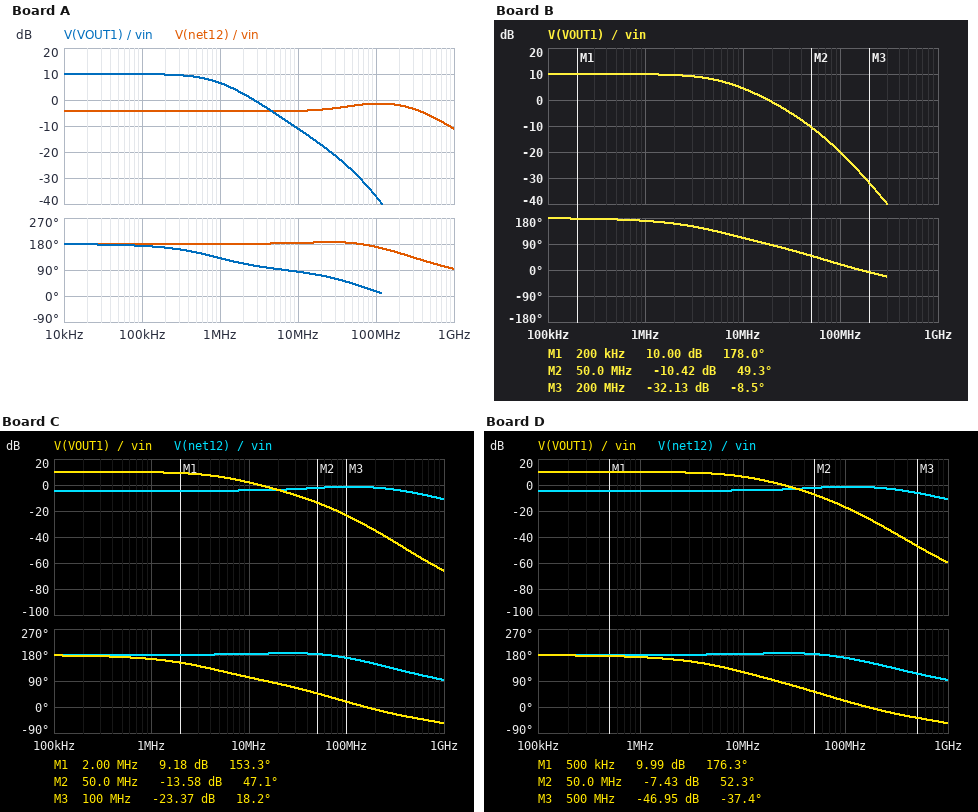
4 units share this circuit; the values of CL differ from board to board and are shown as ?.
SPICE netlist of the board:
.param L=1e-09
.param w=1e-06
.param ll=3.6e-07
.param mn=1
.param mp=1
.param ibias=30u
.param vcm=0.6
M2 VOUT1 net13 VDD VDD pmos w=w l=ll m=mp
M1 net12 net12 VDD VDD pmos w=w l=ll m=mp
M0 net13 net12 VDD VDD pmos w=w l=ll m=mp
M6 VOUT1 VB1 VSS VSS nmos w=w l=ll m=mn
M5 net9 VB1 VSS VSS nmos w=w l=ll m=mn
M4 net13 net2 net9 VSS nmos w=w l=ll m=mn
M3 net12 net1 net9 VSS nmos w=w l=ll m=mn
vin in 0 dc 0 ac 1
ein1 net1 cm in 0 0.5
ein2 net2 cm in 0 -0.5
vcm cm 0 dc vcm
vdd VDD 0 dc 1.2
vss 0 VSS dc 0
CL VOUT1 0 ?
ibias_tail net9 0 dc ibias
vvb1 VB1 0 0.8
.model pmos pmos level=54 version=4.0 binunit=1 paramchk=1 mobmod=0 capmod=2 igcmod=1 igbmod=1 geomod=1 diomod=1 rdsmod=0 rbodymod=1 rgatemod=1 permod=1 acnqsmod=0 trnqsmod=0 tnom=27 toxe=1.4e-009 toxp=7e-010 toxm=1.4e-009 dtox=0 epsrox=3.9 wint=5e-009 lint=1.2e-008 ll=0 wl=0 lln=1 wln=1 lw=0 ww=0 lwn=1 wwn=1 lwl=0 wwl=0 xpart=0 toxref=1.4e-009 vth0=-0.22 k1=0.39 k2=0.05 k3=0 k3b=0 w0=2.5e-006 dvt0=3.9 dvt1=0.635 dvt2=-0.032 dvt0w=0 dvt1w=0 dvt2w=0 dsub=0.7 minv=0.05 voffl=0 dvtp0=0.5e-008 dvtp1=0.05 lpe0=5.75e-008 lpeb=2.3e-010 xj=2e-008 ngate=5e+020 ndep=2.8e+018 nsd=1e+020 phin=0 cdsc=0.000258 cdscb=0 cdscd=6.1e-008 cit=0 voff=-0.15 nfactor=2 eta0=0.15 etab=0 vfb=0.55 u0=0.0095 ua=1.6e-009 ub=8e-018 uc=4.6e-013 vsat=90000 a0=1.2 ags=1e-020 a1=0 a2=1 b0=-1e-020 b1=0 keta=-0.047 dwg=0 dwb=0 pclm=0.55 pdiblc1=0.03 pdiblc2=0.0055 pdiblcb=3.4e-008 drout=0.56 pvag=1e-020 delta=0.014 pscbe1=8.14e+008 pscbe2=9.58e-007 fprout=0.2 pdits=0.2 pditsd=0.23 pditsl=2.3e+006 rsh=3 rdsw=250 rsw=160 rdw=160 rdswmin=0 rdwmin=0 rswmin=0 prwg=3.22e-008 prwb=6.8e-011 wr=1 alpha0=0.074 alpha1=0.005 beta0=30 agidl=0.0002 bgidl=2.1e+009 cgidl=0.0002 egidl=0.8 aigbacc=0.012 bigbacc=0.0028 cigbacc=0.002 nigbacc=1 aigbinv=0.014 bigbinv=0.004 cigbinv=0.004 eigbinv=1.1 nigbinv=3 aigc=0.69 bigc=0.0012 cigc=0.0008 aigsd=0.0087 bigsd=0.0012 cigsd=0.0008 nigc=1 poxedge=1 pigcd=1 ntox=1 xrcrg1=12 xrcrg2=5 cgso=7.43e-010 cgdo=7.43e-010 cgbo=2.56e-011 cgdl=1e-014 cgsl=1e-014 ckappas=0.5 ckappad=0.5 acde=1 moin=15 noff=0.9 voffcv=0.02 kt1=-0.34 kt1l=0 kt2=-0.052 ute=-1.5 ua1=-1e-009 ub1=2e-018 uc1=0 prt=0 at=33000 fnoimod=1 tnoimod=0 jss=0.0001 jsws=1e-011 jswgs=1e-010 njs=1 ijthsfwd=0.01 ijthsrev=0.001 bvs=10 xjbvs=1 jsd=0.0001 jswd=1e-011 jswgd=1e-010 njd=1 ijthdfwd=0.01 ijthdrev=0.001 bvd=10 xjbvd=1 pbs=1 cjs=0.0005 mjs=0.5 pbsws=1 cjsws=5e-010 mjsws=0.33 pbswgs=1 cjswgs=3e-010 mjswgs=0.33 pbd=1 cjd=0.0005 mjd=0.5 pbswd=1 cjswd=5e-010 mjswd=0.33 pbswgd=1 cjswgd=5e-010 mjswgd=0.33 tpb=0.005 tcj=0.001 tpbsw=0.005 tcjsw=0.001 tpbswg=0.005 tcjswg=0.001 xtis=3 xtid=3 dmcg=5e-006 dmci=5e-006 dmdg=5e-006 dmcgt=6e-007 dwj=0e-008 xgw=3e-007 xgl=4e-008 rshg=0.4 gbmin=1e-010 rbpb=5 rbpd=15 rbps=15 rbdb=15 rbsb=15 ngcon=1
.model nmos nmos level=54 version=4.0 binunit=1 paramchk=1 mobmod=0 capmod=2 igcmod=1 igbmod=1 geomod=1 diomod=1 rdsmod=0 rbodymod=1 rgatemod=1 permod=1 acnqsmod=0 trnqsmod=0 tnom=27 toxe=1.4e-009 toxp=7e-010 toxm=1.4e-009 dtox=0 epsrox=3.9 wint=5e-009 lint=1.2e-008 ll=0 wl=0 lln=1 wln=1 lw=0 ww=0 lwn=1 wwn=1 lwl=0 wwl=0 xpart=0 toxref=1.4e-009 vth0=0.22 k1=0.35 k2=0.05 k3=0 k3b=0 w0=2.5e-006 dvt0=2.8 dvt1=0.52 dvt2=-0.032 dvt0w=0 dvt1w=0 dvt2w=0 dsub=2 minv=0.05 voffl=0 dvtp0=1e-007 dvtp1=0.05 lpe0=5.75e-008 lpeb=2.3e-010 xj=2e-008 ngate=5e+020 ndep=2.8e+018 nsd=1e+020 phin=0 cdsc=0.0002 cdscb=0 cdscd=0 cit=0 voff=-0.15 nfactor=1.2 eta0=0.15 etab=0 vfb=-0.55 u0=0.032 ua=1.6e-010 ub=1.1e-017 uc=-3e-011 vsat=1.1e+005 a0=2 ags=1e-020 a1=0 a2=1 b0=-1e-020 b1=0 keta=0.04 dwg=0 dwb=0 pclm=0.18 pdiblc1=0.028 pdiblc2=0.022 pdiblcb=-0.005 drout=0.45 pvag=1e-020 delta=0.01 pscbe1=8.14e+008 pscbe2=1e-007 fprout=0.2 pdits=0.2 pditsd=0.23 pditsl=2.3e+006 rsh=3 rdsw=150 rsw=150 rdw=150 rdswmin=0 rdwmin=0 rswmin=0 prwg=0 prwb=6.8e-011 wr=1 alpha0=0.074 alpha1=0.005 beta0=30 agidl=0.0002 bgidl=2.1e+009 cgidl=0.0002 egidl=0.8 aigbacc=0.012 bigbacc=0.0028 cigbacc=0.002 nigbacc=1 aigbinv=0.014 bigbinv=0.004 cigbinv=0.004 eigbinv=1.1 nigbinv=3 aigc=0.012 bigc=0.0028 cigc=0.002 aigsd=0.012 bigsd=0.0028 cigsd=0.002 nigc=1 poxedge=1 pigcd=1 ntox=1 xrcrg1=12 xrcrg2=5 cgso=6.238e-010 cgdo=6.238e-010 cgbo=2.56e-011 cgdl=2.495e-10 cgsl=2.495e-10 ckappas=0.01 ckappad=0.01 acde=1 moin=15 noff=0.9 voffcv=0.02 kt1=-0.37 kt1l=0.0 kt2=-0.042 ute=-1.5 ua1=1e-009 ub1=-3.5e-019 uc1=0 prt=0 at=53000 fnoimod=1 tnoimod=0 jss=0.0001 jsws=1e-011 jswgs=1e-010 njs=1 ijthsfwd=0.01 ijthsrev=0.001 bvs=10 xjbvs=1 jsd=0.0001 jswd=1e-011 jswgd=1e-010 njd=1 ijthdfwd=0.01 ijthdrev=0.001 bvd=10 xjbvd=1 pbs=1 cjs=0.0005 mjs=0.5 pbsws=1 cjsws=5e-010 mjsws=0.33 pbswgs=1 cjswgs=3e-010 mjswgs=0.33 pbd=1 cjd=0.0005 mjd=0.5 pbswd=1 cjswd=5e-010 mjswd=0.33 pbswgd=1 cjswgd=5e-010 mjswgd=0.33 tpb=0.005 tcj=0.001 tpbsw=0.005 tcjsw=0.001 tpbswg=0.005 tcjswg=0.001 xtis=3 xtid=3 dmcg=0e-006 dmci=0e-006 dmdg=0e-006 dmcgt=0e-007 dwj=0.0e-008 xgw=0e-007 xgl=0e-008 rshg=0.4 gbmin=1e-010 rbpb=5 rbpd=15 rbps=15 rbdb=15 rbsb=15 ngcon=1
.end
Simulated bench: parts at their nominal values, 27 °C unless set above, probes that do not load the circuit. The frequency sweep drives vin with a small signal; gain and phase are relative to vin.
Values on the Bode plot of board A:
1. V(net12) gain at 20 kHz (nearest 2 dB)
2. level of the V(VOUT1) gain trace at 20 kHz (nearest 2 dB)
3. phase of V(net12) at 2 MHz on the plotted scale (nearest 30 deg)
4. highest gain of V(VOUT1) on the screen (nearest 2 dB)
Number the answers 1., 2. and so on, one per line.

1. -4 dB
2. 10 dB
3. 180 deg
4. 10 dB
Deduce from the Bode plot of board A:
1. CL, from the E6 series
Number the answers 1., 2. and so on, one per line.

1. 33 pF
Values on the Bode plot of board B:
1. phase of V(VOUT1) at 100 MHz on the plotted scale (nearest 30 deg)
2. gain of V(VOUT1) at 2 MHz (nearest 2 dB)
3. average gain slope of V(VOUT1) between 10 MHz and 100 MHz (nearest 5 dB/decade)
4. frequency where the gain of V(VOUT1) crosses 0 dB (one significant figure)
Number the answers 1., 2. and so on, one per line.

1. 30 deg
2. 10 dB
3. -25 dB/decade
4. 20 MHz
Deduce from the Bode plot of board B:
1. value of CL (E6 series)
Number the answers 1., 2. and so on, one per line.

1. 4.7 pF
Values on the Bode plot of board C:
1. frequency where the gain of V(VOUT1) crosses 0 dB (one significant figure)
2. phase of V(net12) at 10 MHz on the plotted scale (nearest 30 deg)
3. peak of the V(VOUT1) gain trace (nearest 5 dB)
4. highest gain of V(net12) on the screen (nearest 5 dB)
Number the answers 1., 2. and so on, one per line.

1. 10 MHz
2. 180 deg
3. 10 dB
4. 0 dB
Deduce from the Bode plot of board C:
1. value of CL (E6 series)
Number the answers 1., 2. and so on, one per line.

1. 6.8 pF
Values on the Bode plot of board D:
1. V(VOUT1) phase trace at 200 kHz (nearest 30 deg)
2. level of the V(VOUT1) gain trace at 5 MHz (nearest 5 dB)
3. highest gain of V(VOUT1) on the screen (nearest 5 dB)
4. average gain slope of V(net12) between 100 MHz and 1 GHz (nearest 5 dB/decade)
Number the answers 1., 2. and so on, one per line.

1. 180 deg
2. 10 dB
3. 10 dB
4. -10 dB/decade
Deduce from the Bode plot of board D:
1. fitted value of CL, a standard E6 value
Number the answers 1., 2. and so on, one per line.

1. 3.3 pF
